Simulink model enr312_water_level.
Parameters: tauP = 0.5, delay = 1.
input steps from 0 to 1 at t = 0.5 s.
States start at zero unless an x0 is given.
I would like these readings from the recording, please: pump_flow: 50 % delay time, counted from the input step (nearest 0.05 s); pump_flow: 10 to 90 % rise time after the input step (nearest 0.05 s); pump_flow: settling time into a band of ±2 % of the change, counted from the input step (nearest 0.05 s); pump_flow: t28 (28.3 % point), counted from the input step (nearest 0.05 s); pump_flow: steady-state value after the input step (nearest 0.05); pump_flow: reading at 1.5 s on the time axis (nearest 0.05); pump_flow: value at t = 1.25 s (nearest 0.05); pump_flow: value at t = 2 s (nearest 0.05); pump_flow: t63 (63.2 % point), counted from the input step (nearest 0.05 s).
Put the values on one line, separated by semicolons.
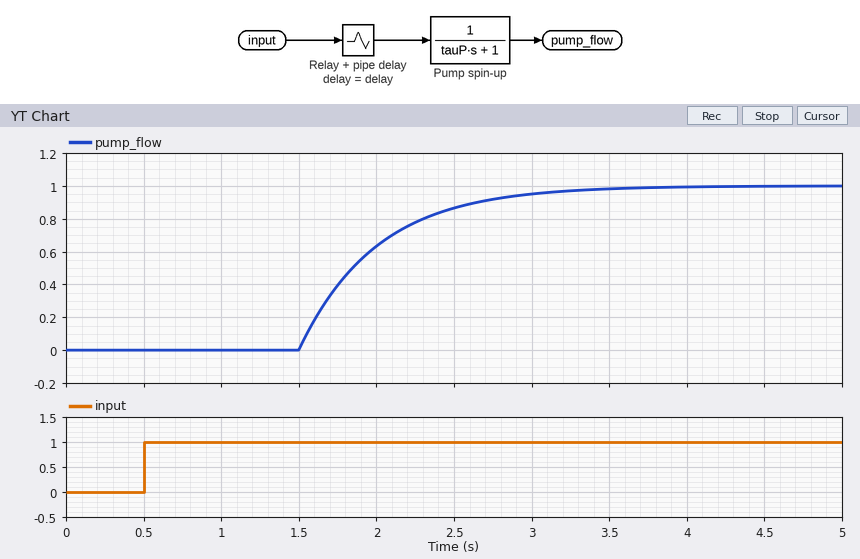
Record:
1.35 s; 1.10 s; 2.95 s; 1.15 s; 1.00; 0.00; 0.00; 0.65; 1.50 s
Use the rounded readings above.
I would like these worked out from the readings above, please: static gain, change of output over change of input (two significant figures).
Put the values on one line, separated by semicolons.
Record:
1.0
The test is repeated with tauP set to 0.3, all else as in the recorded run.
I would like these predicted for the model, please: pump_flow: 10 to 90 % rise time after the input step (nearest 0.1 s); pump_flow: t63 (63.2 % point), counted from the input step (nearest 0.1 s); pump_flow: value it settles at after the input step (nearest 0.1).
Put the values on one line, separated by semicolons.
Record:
0.7 s; 1.3 s; 1.0
